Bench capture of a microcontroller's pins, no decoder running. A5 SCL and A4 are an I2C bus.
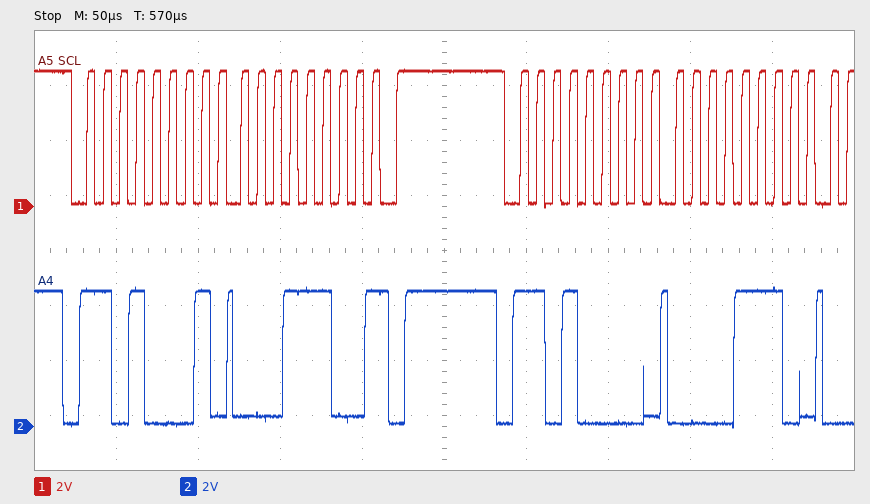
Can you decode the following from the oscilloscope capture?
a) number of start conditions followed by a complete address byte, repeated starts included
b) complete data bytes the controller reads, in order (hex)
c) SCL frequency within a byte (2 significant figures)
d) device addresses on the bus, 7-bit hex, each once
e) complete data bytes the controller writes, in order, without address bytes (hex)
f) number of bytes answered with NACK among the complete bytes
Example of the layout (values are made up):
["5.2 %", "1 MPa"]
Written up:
["2", "1C", "100 kHz", "0x68", "0E", "1"]
